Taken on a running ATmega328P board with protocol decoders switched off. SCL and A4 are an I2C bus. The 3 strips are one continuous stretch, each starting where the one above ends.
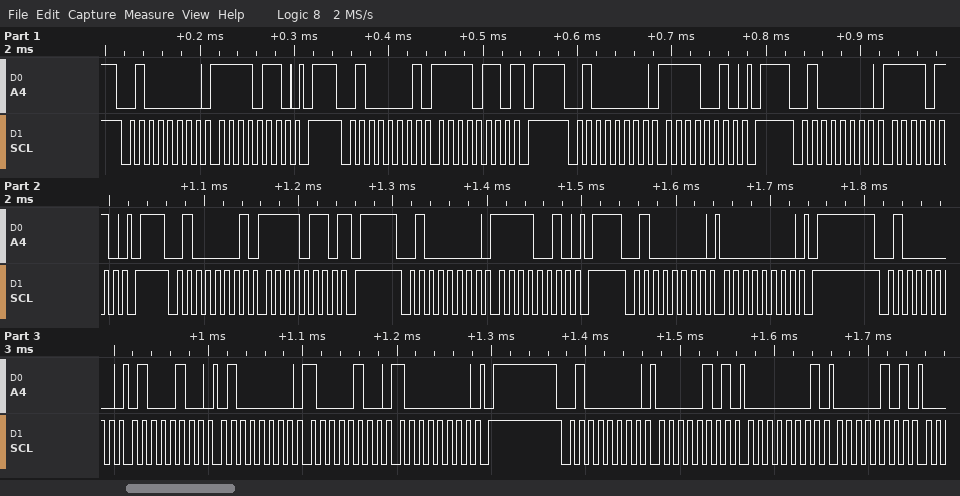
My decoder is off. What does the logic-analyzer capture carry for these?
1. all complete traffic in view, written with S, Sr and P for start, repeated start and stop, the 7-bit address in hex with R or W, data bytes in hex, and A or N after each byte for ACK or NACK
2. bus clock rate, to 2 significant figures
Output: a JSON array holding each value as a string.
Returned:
["S 20W A F6 A P S 20R A F6 N P S 20W A F2 A P S 20W A F6 A P S 20R A F6 N P S 20W A F2 A P S 20W A 00 A P S 20W A 44 A 40 A 84 A 80 A P S 20W A 05 A 01 A 05 A", "100 kHz"]
